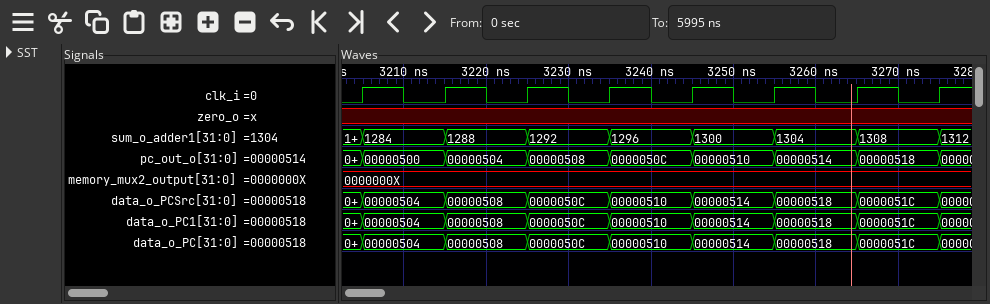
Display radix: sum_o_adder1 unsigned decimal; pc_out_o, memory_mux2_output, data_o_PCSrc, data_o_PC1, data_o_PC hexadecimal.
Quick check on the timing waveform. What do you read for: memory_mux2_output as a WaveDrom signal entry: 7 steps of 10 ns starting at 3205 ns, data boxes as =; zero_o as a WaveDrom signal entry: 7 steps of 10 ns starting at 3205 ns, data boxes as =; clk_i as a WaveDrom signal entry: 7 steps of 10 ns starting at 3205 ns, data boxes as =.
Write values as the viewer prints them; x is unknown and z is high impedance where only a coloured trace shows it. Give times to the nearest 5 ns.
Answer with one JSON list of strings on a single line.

["{name: 'memory_mux2_output', wave: '=......', data: '0000000X'}", "{name: 'zero_o', wave: 'x......'}", "{name: 'clk_i', wave: 'p......'}"]
